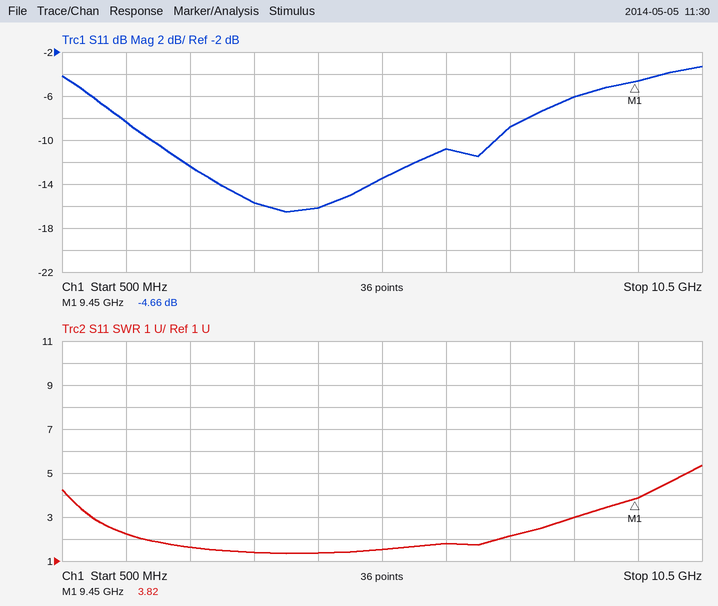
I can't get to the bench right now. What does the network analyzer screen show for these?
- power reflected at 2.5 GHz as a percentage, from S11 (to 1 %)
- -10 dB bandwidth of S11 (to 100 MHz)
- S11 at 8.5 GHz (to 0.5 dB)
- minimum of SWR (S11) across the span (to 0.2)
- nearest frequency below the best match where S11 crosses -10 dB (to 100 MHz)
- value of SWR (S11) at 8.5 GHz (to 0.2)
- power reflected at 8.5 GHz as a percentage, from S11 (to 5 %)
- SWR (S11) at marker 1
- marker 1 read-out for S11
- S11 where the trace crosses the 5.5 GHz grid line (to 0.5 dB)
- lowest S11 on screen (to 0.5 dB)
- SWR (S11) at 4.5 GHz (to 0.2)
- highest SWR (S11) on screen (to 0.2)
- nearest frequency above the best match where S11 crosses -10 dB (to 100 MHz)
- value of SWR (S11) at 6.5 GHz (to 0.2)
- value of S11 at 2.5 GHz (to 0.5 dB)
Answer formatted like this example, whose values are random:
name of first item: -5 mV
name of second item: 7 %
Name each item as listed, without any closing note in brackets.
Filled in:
power reflected at 2.5 GHz as a percentage, from S11: 6 %
-10 dB bandwidth of S11: 5.4 GHz
S11 at 8.5 GHz: -6.0 dB
minimum of SWR (S11) across the span: 1.4
nearest frequency below the best match where S11 crosses -10 dB: 1.9 GHz
value of SWR (S11) at 8.5 GHz: 3.0
power reflected at 8.5 GHz as a percentage, from S11: 25 %
SWR (S11) at marker 1: 3.82
marker 1 read-out for S11: -4.66 dB
S11 where the trace crosses the 5.5 GHz grid line: -13.5 dB
lowest S11 on screen: -16.5 dB
SWR (S11) at 4.5 GHz: 1.4
highest SWR (S11) on screen: 5.4
nearest frequency above the best match where S11 crosses -10 dB: 7.3 GHz
value of SWR (S11) at 6.5 GHz: 1.8
value of S11 at 2.5 GHz: -12.5 dB
